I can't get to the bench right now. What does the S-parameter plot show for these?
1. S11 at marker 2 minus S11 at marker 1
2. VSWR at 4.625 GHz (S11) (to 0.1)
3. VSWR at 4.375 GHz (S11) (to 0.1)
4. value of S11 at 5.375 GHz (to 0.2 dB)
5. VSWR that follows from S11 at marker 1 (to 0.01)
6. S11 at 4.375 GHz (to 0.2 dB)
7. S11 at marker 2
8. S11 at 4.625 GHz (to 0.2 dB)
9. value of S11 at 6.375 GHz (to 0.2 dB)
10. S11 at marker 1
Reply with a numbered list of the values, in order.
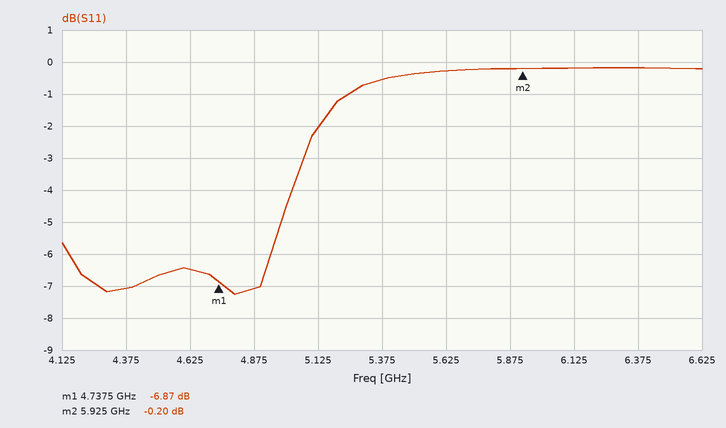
1. 6.67 dB
2. 2.8
3. 2.6
4. -0.6 dB
5. 2.66
6. -7.0 dB
7. -0.20 dB
8. -6.4 dB
9. -0.2 dB
10. -6.87 dB
